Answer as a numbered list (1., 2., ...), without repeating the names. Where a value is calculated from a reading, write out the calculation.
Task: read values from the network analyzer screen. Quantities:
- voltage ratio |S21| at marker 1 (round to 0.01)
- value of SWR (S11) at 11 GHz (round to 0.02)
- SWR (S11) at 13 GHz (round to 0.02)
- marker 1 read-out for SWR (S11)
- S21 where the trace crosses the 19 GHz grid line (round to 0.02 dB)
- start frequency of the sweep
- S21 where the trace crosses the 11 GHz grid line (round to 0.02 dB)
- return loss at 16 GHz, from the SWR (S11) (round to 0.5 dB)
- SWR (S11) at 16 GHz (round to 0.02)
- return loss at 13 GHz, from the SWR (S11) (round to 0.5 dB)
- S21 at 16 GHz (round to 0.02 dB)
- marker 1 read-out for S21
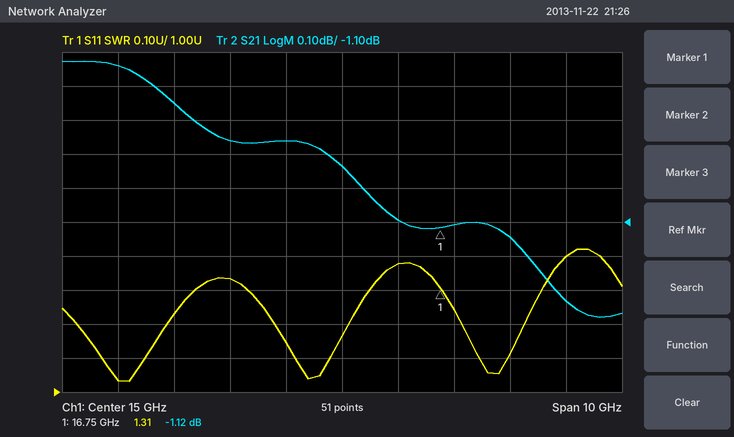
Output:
1. 10^(-1.12/20) ≈ 0.88
2. 1.04
3. 1.34
4. 1.31
5. -1.34 dB
6. 10 GHz
7. -0.64 dB
8. −20 log10((1.38 − 1)/(1.38 + 1)) ≈ 15.9 dB, so 16.0 dB to the nearest 0.5 dB
9. 1.38
10. −20 log10((1.34 − 1)/(1.34 + 1)) ≈ 16.8 dB, so 17.0 dB to the nearest 0.5 dB
11. -1.10 dB
12. -1.12 dB
